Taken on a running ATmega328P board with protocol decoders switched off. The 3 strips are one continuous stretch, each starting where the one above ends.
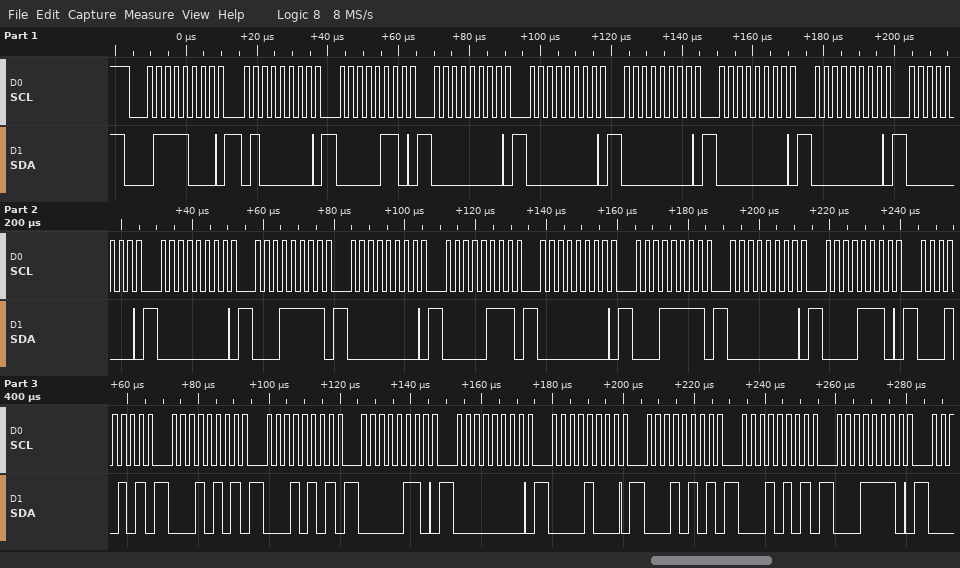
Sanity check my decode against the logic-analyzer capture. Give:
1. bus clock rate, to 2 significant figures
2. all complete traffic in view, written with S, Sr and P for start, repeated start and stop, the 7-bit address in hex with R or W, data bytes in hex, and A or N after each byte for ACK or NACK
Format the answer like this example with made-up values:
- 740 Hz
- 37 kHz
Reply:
- 400 kHz
- S 3CW A 40 A 06 A 00 A 00 A 00 A 00 A 00 A 00 A 00 A 1F A 00 A 07 A 00 A 1F A 00 A 0E A 15 A 15 A 15 A 06 A 00 A 08 A 15 A 15 A 1E A
